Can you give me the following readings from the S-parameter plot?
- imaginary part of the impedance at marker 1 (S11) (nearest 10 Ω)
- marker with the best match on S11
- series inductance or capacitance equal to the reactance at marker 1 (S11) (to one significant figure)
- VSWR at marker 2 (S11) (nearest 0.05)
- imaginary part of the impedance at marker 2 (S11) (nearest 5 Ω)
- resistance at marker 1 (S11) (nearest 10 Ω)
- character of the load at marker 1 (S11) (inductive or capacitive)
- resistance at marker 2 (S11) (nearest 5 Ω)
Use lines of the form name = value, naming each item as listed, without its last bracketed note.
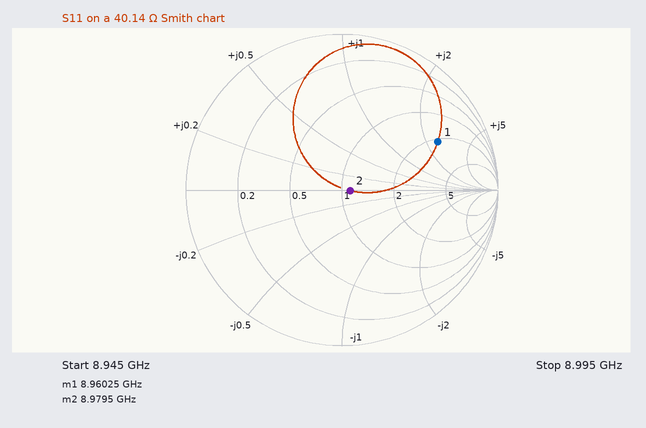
imaginary part of the impedance at marker 1 (S11) = +100 Ω
marker with the best match on S11 = marker 2
series inductance or capacitance equal to the reactance at marker 1 (S11) = 2 nH
VSWR at marker 2 (S11) = 1.10
imaginary part of the impedance at marker 2 (S11) = 0 Ω
resistance at marker 1 (S11) = 90 Ω
character of the load at marker 1 (S11) = inductive
resistance at marker 2 (S11) = 45 Ω
